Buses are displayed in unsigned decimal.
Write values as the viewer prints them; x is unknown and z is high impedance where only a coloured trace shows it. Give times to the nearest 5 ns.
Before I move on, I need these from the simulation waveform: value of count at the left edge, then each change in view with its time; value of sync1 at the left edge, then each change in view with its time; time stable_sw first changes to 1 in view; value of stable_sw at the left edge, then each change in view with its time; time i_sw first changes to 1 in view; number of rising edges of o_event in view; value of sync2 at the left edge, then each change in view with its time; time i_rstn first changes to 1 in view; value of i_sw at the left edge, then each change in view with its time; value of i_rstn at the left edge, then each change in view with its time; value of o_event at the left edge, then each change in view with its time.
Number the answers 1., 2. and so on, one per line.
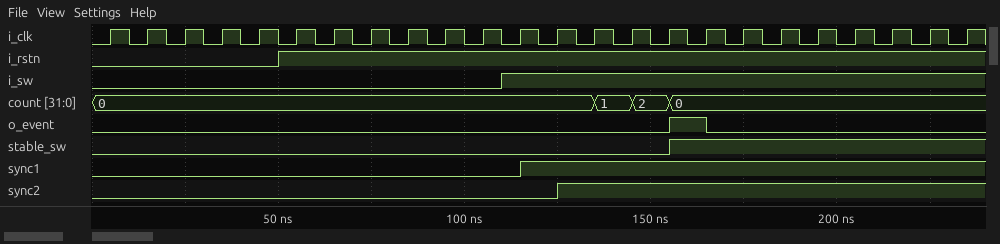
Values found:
1. 0, 1 at 135 ns, 2 at 145 ns, 0 at 155 ns
2. 0, 1 at 115 ns
3. 155 ns
4. 0, 1 at 155 ns
5. 110 ns
6. 1
7. 0, 1 at 125 ns
8. 50 ns
9. 0, 1 at 110 ns
10. 0, 1 at 50 ns
11. 0, 1 at 155 ns, 0 at 165 ns
